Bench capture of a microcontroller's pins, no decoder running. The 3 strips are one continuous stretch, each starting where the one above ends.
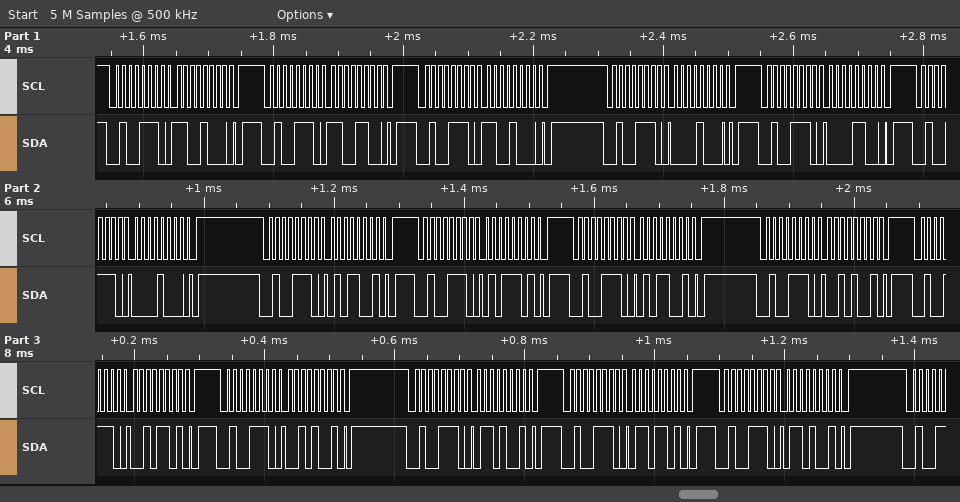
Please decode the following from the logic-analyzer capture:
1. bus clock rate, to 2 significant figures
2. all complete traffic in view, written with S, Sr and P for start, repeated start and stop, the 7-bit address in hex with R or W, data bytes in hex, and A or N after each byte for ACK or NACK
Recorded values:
100 kHz
S 27W A C8 A P S 27W A CC A P S 27W A C8 A P S 27W A 08 A P S 27W A 0C A P S 27W A 08 A P S 27W A 59 A P S 27W A 5D A P S 27W A 59 A P S 27W A 29 A P S 27W A 2D A P S 27W A 29 A P S 27W A 69 A P S 27W A 6D A P S 27W A 69 A P
